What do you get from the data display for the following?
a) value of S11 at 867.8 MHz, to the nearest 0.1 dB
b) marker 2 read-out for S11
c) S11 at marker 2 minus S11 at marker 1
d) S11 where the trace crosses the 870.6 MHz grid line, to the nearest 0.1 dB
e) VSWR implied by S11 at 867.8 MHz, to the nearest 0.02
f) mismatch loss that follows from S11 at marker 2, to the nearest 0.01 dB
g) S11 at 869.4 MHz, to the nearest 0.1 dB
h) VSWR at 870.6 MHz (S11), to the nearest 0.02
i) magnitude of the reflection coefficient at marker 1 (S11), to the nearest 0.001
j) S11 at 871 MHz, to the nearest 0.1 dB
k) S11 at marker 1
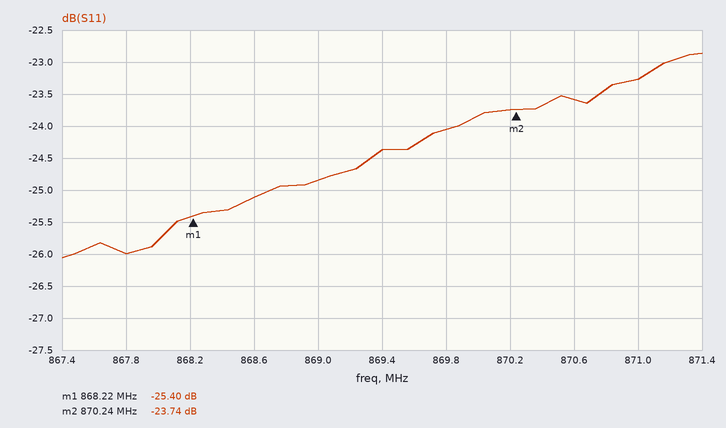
-26.0 dB
-23.74 dB
1.66 dB
-23.6 dB
1.10
0.02 dB
-24.4 dB
1.14
0.054
-23.3 dB
-25.40 dB
